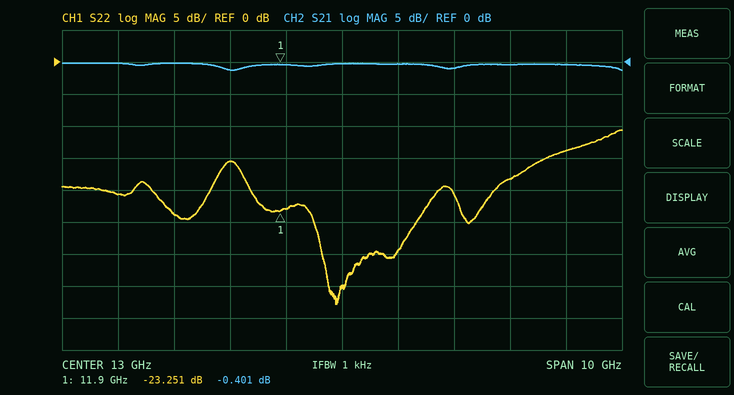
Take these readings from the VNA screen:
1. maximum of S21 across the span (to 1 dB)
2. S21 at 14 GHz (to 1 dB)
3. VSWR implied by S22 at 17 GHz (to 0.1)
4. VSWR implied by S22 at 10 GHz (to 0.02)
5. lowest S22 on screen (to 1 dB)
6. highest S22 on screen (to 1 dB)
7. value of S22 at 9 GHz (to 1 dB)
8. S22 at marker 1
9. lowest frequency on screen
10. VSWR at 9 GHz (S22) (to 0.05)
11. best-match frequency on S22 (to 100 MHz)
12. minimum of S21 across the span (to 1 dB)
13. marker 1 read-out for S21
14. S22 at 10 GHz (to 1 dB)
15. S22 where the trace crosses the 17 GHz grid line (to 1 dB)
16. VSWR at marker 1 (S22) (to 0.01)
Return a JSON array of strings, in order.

["0 dB", "0 dB", "1.5", "1.14", "-38 dB", "-11 dB", "-21 dB", "-23.251 dB", "8 GHz", "1.20", "12.9 GHz", "-1 dB", "-0.401 dB", "-24 dB", "-14 dB", "1.15"]
